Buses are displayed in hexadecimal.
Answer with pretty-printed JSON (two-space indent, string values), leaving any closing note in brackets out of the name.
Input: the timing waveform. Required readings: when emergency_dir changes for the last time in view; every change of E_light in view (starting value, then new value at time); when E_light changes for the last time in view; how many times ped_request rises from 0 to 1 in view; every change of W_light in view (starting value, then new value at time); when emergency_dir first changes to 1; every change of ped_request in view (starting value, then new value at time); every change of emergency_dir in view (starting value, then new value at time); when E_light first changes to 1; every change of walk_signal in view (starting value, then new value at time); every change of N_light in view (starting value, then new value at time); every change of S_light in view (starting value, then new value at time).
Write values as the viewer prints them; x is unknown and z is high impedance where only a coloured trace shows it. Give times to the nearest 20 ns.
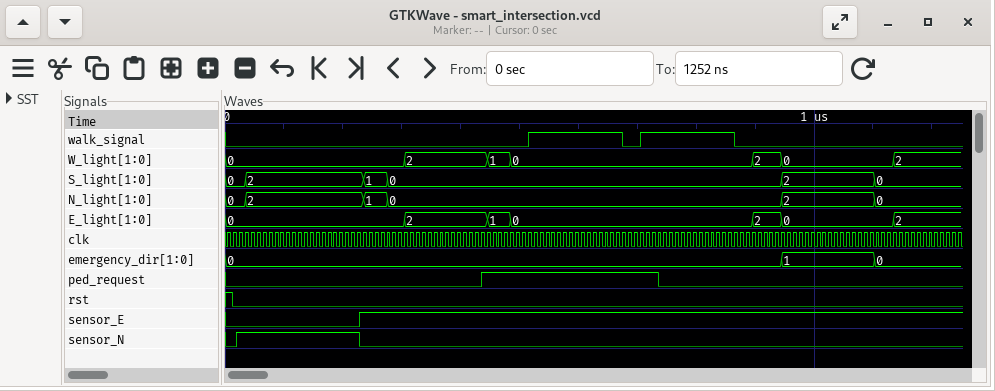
{
  "when emergency_dir changes for the last time in view": "1100 ns",
  "every change of E_light in view": "0, 2 at 300 ns, 1 at 440 ns, 0 at 480 ns, 2 at 900 ns, 0 at 940 ns, 2 at 1140 ns",
  "when E_light changes for the last time in view": "1140 ns",
  "how many times ped_request rises from 0 to 1 in view": "1",
  "every change of W_light in view": "0, 2 at 300 ns, 1 at 440 ns, 0 at 480 ns, 2 at 900 ns, 0 at 940 ns, 2 at 1140 ns",
  "when emergency_dir first changes to 1": "940 ns",
  "every change of ped_request in view": "0, 1 at 440 ns, 0 at 740 ns",
  "every change of emergency_dir in view": "0, 1 at 940 ns, 0 at 1100 ns",
  "when E_light first changes to 1": "440 ns",
  "every change of walk_signal in view": "0, 1 at 520 ns, 0 at 680 ns, 1 at 700 ns, 0 at 860 ns",
  "every change of N_light in view": "0, 2 at 40 ns, 1 at 240 ns, 0 at 280 ns, 2 at 940 ns, 0 at 1100 ns",
  "every change of S_light in view": "0, 2 at 40 ns, 1 at 240 ns, 0 at 280 ns, 2 at 940 ns, 0 at 1100 ns"
}
